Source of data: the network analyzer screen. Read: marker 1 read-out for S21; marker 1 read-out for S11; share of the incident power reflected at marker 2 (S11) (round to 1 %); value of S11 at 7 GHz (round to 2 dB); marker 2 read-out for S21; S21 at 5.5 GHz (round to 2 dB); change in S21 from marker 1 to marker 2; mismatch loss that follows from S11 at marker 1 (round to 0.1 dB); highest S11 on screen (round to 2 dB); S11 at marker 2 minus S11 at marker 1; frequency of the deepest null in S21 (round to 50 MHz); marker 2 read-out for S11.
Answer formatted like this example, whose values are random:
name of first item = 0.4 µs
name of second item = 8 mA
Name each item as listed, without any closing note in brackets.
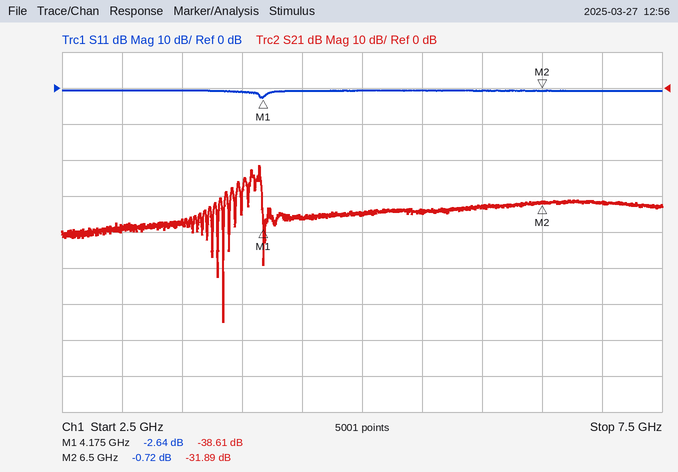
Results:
marker 1 read-out for S21 = -38.61 dB
marker 1 read-out for S11 = -2.64 dB
share of the incident power reflected at marker 2 (S11) = 85 %
value of S11 at 7 GHz = 0 dB
marker 2 read-out for S21 = -31.89 dB
S21 at 5.5 GHz = -34 dB
change in S21 from marker 1 to marker 2 = 6.72 dB
mismatch loss that follows from S11 at marker 1 = 3.4 dB
highest S11 on screen = 0 dB
S11 at marker 2 minus S11 at marker 1 = 1.92 dB
frequency of the deepest null in S21 = 3.85 GHz
marker 2 read-out for S11 = -0.72 dB
